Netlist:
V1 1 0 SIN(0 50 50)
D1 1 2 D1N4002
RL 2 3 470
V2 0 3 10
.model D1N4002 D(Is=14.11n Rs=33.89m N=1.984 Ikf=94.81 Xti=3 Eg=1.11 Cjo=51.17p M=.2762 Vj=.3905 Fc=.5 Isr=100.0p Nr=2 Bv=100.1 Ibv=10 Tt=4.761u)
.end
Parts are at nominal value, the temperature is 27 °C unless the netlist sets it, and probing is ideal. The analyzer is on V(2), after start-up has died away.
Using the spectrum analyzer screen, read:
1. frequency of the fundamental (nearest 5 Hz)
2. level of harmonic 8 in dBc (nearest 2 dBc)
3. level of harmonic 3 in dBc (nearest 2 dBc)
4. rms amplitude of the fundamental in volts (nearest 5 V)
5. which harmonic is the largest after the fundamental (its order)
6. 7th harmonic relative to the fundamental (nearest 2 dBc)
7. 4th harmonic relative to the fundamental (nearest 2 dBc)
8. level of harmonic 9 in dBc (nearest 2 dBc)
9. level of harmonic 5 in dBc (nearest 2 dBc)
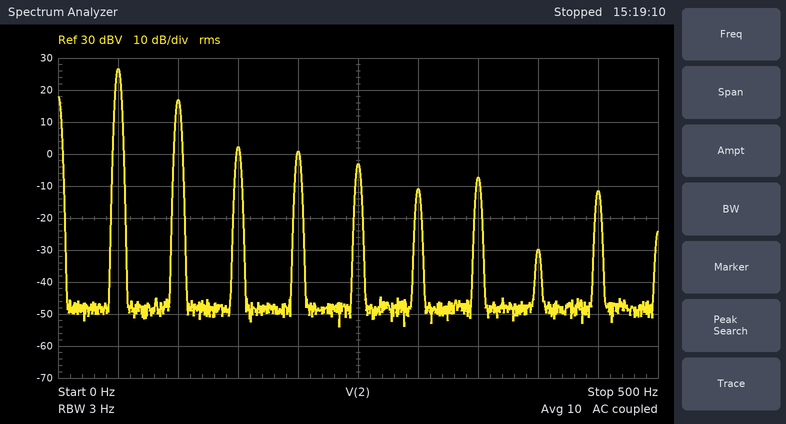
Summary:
50 Hz
-56 dBc
-24 dBc
20 V
2
-34 dBc
-26 dBc
-38 dBc
-30 dBc
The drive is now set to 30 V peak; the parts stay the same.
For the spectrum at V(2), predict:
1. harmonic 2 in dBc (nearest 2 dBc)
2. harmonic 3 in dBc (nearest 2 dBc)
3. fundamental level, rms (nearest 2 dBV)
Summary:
-12 dBc
-22 dBc
24 dBV
